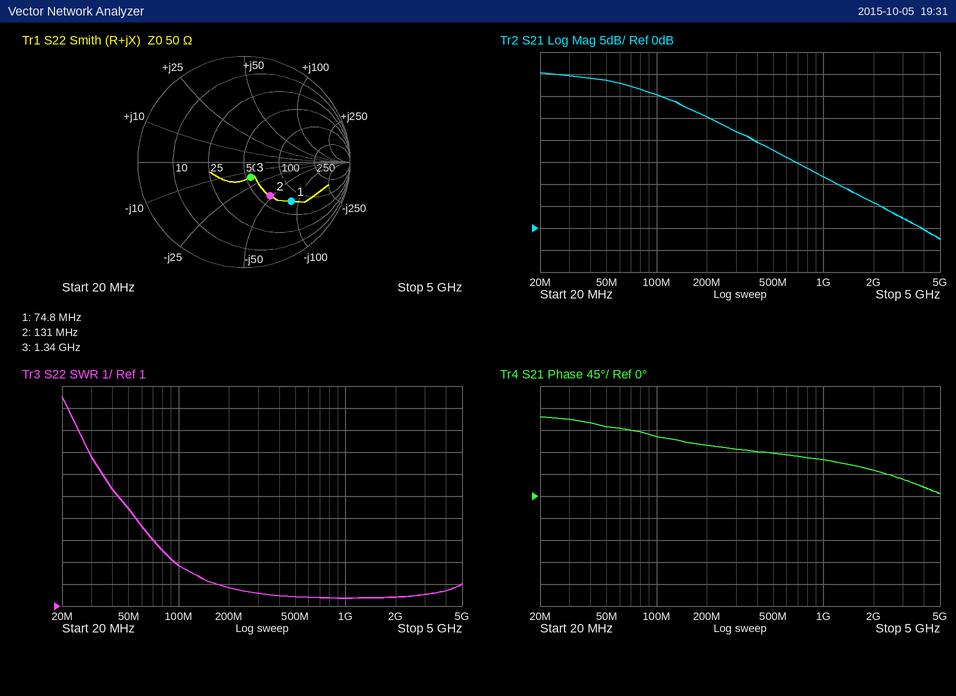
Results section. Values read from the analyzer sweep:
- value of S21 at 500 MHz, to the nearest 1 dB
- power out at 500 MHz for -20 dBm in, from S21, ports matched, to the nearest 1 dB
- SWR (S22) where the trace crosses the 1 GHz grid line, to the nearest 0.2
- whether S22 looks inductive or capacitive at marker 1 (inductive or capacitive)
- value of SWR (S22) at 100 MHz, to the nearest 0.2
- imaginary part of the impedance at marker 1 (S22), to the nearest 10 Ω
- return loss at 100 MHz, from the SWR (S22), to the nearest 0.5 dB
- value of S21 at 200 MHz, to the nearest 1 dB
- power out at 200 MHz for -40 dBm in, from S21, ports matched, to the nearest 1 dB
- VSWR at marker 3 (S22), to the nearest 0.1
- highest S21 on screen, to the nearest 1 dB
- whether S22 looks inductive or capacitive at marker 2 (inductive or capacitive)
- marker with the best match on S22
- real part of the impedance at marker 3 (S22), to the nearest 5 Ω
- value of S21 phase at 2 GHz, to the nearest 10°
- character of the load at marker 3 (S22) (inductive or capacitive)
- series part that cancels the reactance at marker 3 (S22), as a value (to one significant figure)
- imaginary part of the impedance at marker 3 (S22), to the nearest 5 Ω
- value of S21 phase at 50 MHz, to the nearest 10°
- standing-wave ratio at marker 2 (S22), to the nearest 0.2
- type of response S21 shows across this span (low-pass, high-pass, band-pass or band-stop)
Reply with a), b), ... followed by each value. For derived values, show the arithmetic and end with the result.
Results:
a) 18 dB
b) -20 dBm + (18 dB) = -2 dBm
c) 1.4
d) capacitive
e) 2.8
f) -80 Ω
g) −20 log10((2.8 − 1)/(2.8 + 1)) ≈ 6.5 dB
h) 25 dB
i) -40 dBm + (25 dB) = -15 dBm
j) 1.4
k) 35 dB
l) capacitive
m) marker 3
n) 55 Ω
o) 50°
p) capacitive
q) L = 15 Ω/(2π × 1.34 GHz) ≈ 2 nH
r) -15 Ω
s) 140°
t) 2.4
u) low-pass
